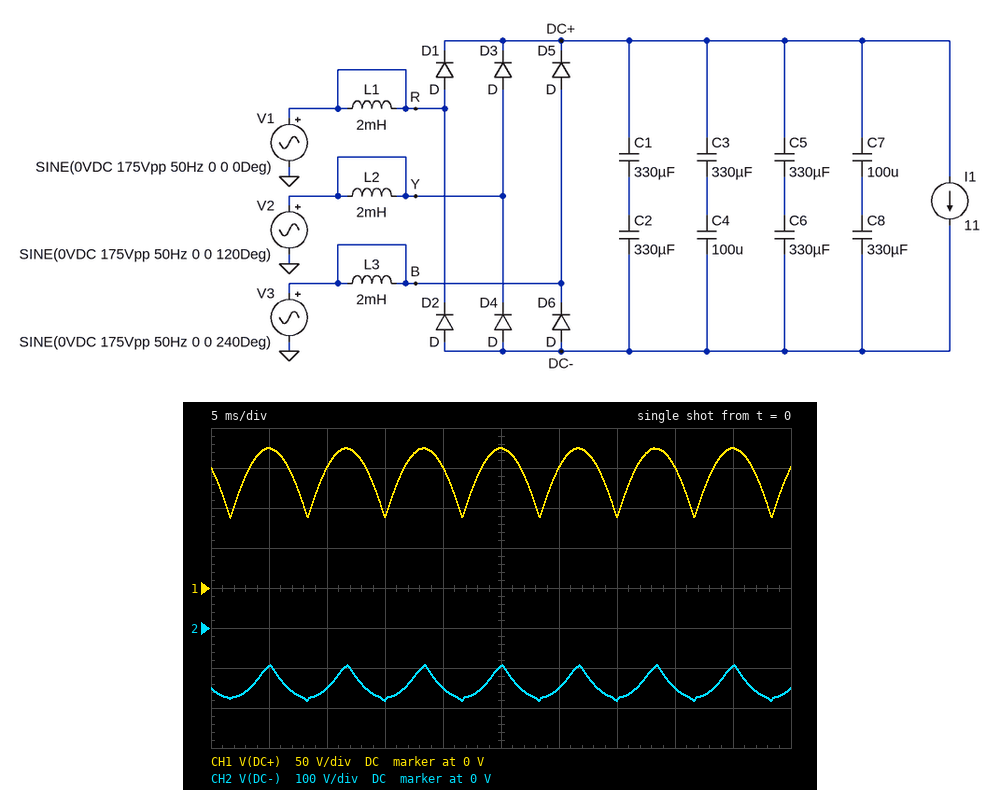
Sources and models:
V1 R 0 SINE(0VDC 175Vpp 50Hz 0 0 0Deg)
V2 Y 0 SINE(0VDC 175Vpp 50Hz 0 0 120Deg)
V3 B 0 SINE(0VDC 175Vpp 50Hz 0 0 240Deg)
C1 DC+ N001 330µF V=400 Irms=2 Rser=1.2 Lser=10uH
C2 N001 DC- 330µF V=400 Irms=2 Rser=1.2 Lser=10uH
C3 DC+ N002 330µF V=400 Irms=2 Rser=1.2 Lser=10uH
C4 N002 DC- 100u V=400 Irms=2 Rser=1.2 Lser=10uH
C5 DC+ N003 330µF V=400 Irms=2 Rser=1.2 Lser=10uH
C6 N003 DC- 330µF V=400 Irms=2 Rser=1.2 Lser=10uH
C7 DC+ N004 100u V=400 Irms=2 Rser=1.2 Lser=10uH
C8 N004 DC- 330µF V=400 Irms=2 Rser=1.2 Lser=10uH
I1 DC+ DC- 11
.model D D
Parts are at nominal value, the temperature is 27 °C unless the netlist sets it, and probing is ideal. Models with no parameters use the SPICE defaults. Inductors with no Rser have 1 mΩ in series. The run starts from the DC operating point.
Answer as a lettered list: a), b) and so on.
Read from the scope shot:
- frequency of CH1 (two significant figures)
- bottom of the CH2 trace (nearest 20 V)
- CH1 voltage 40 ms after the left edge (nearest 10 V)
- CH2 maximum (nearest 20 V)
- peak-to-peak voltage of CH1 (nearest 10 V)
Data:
a) 150 Hz
b) -180 V
c) 150 V
d) -100 V
e) 90 V
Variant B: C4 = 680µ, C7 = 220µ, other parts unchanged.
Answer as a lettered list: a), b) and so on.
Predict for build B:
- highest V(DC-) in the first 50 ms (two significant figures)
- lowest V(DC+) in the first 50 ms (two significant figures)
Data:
a) -98 V
b) 89 V
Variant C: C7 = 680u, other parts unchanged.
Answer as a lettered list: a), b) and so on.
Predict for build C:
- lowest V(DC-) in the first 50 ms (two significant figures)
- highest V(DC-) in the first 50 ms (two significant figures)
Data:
a) -190 V
b) -97 V
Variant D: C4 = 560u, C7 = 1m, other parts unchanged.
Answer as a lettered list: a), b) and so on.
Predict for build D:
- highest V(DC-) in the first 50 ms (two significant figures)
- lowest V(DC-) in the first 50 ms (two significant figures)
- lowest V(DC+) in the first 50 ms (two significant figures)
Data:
a) -100 V
b) -190 V
c) 87 V
